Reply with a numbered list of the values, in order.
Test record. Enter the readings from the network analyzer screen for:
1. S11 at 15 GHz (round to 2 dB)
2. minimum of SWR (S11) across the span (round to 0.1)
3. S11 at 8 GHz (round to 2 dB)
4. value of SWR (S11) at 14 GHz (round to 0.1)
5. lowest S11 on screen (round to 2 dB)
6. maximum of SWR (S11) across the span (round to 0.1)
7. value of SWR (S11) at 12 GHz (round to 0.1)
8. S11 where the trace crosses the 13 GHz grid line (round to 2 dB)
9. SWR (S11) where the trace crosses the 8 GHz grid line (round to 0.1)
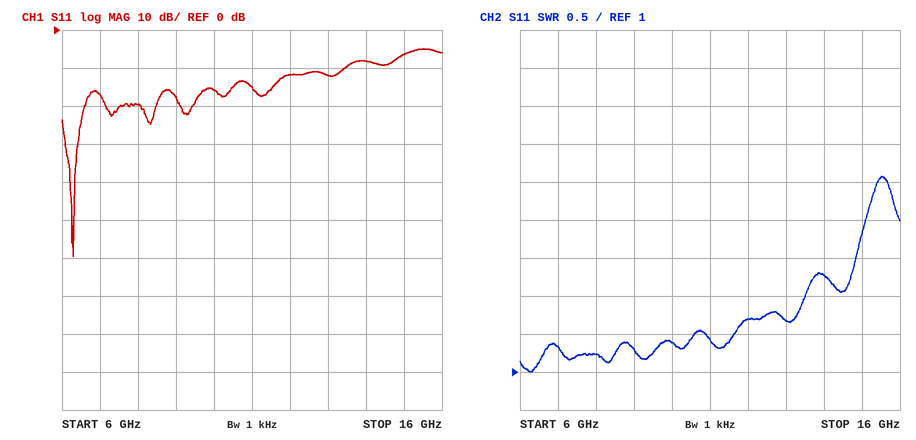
1. -6 dB
2. 1.0
3. -20 dB
4. 2.3
5. -60 dB
6. 3.6
7. 1.7
8. -12 dB
9. 1.2
